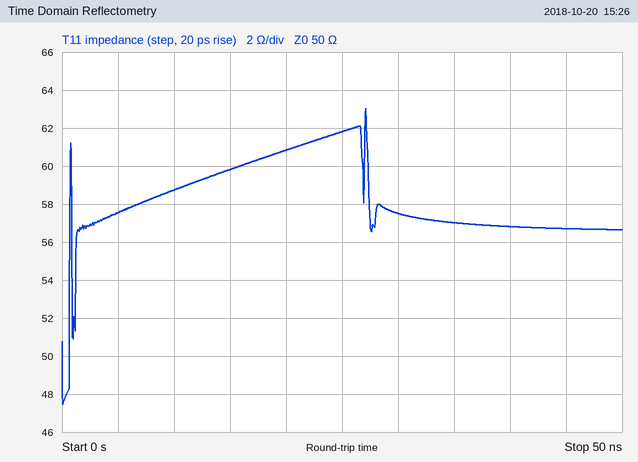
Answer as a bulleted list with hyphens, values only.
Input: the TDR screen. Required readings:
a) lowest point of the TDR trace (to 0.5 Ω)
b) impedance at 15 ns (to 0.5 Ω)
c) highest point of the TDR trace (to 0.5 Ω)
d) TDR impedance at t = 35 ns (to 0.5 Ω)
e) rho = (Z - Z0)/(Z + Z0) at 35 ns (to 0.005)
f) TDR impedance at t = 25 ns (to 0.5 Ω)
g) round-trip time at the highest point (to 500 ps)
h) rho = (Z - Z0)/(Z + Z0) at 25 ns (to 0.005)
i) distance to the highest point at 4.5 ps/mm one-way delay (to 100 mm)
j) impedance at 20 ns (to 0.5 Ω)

- 47.5 Ω
- 60.0 Ω
- 63.0 Ω
- 57.0 Ω
- +0.065
- 62.0 Ω
- 27.0 ns
- +0.105
- 3.0 m
- 61.0 Ω
